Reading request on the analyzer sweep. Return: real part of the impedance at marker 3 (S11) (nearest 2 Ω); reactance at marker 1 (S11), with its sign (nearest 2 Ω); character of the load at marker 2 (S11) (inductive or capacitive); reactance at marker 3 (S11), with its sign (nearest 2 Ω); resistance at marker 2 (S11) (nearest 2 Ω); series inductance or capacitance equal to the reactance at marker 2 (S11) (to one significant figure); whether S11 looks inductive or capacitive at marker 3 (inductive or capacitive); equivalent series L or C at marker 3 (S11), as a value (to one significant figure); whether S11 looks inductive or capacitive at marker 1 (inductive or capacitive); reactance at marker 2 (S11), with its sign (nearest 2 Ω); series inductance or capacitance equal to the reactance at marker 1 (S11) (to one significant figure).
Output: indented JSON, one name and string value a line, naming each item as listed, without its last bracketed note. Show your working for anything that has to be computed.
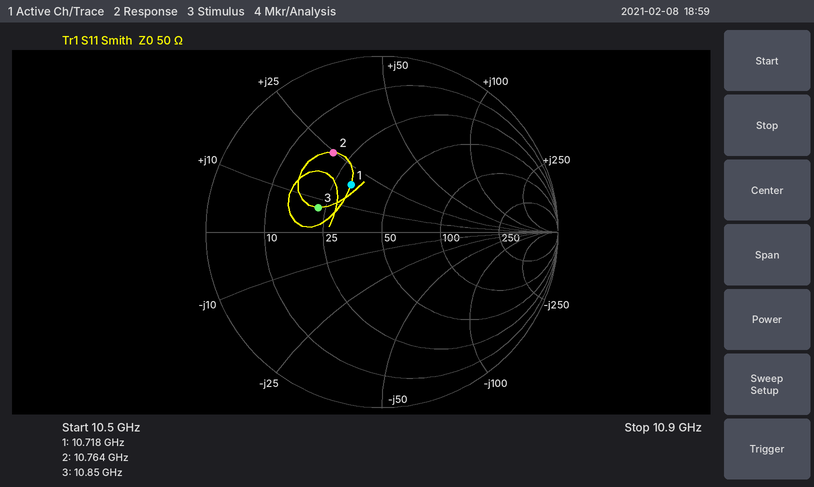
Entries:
{
  "real part of the impedance at marker 3 (S11)": "22 Ω",
  "reactance at marker 1 (S11), with its sign": "+18 Ω",
  "character of the load at marker 2 (S11)": "inductive",
  "reactance at marker 3 (S11), with its sign": "+8 Ω",
  "resistance at marker 2 (S11)": "20 Ω",
  "series inductance or capacitance equal to the reactance at marker 2 (S11)": "L = 24 Ω/(2π × 10.764 GHz) ≈ 355 pH, so 400 pH to one significant figure",
  "whether S11 looks inductive or capacitive at marker 3": "inductive",
  "equivalent series L or C at marker 3 (S11), as a value": "L = 8 Ω/(2π × 10.85 GHz) ≈ 117 pH, so 100 pH to one significant figure",
  "whether S11 looks inductive or capacitive at marker 1": "inductive",
  "reactance at marker 2 (S11), with its sign": "+24 Ω",
  "series inductance or capacitance equal to the reactance at marker 1 (S11)": "L = 18 Ω/(2π × 10.718 GHz) ≈ 267 pH, so 300 pH to one significant figure"
}
